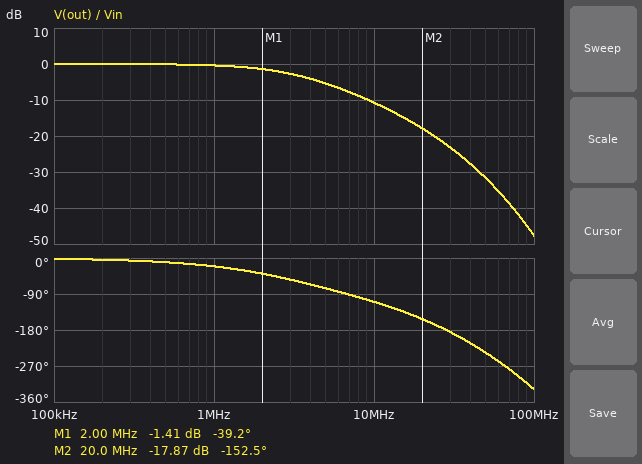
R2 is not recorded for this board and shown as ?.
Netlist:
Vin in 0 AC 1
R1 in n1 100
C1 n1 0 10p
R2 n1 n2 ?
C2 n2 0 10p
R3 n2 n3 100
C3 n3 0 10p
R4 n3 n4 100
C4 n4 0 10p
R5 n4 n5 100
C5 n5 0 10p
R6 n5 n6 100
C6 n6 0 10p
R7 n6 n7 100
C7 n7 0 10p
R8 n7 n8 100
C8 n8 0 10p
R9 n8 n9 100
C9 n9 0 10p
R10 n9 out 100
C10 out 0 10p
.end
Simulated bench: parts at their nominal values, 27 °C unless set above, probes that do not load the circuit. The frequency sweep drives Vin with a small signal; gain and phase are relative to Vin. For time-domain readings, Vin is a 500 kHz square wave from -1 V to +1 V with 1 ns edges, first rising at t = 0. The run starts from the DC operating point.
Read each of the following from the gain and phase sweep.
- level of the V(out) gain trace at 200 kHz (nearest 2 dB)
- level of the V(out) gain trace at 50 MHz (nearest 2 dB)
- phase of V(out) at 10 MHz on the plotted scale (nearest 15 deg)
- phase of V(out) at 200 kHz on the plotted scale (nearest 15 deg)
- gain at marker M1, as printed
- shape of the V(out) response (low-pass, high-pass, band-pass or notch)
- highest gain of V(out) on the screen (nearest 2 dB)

0 dB
-32 dB
-105 deg
0 deg
-1.41 dB
low-pass
0 dB
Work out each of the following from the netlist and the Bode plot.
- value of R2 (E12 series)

150 Ω
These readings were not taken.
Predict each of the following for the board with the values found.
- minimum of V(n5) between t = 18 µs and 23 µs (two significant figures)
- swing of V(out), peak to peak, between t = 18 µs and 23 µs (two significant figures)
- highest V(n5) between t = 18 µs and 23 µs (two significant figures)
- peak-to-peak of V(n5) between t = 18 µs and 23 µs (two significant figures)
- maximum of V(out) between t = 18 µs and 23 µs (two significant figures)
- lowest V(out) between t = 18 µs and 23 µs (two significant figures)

-1.0 V
2.0 V
1.0 V
2.0 V
1.0 V
-1.0 V
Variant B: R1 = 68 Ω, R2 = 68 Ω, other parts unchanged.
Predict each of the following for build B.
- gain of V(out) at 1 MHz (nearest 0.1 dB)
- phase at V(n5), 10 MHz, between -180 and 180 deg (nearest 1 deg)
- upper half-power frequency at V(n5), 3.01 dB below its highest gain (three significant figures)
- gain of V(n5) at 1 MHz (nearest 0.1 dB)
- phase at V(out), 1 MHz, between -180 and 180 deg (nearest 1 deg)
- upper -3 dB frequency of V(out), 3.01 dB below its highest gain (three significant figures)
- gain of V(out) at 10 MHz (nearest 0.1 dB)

-0.3 dB
-54 deg
4.40 MHz
-0.2 dB
-17 deg
3.96 MHz
-9.0 dB
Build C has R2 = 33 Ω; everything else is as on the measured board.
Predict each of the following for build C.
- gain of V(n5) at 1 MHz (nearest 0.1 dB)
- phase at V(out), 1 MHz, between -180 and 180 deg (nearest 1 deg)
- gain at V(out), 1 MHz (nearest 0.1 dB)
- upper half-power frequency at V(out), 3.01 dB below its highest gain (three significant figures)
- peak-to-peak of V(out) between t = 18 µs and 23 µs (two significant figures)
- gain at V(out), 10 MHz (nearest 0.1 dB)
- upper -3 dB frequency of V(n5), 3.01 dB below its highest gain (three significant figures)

-0.2 dB
-17 deg
-0.3 dB
3.97 MHz
2.0 V
-9.0 dB
4.41 MHz
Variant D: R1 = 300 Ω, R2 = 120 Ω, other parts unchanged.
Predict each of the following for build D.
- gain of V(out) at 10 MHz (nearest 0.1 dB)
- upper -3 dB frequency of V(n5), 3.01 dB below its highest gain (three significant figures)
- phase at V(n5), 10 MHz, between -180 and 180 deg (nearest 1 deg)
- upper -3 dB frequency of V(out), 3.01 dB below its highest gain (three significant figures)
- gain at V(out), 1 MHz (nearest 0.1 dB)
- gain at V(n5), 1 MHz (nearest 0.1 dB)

-13.2 dB
2.54 MHz
-72 deg
2.44 MHz
-0.7 dB
-0.6 dB
